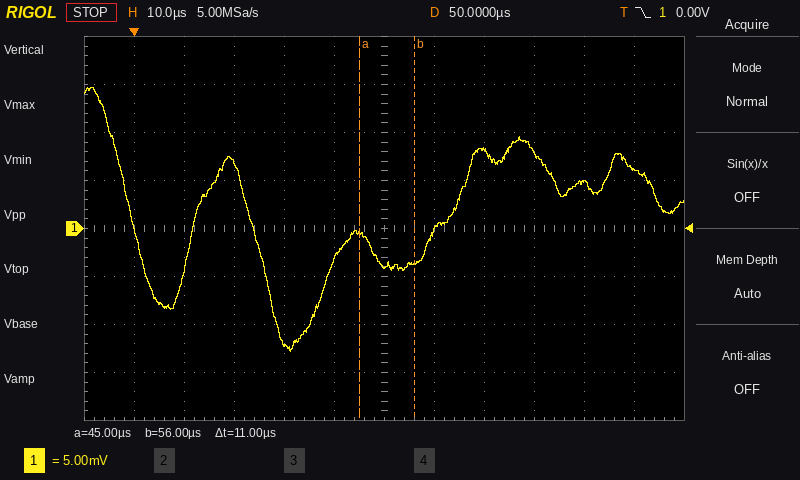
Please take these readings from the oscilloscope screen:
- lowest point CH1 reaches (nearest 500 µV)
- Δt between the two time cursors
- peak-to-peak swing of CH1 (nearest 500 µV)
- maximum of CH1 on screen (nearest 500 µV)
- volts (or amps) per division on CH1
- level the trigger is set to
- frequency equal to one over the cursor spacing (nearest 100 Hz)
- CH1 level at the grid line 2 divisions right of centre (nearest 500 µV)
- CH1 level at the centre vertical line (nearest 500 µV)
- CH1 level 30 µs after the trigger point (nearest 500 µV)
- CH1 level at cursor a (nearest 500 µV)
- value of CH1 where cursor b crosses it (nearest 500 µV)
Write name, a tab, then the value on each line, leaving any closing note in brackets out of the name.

lowest point CH1 reaches	-13.0 mV
Δt between the two time cursors	11 µs
peak-to-peak swing of CH1	27.5 mV
maximum of CH1 on screen	14.5 mV
volts (or amps) per division on CH1	5 mV
level the trigger is set to	0.00 V
frequency equal to one over the cursor spacing	90.9 kHz
CH1 level at the grid line 2 divisions right of centre	8.0 mV
CH1 level at the centre vertical line	-4.0 mV
CH1 level 30 µs after the trigger point	-12.0 mV
CH1 level at cursor a	-500 µV
value of CH1 where cursor b crosses it	-3.5 mV
